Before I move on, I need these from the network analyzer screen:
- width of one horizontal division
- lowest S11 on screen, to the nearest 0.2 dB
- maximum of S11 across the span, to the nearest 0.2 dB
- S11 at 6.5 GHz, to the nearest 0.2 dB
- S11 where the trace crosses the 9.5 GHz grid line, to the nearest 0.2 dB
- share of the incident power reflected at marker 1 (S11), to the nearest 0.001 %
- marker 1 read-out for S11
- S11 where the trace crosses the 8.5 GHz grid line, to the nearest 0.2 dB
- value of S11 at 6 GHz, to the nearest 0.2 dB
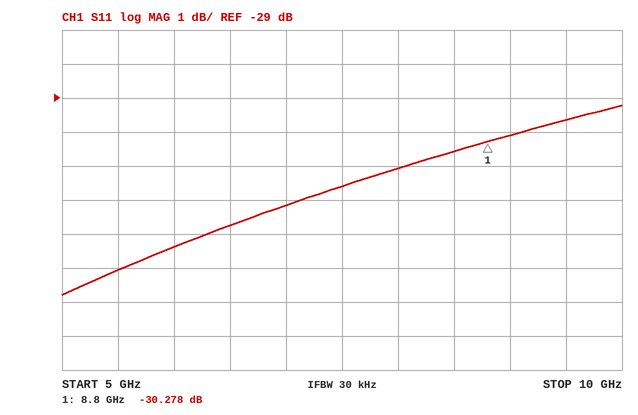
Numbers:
500 MHz
-34.8 dB
-29.2 dB
-32.8 dB
-29.6 dB
0.094 %
-30.278 dB
-30.6 dB
-33.4 dB
